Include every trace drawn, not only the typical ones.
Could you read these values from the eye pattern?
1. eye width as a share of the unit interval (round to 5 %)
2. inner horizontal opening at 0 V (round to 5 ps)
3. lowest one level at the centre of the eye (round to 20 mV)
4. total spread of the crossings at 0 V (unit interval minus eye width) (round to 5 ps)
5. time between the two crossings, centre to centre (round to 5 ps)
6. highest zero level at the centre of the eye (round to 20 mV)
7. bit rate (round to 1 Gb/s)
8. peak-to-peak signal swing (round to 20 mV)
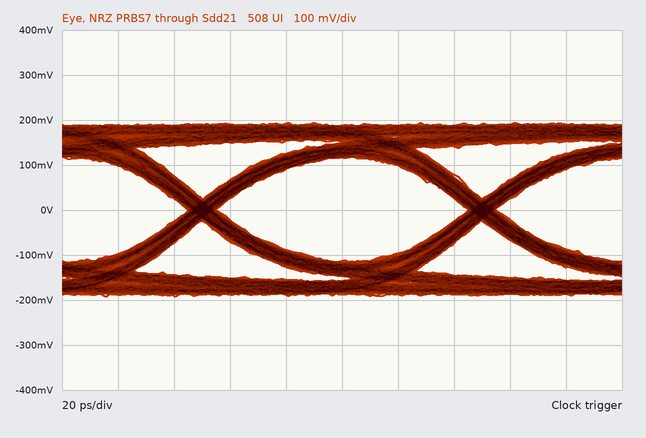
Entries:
90 %
90 ps
120 mV
10 ps
100 ps
-120 mV
10 Gb/s
380 mV
